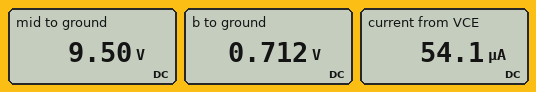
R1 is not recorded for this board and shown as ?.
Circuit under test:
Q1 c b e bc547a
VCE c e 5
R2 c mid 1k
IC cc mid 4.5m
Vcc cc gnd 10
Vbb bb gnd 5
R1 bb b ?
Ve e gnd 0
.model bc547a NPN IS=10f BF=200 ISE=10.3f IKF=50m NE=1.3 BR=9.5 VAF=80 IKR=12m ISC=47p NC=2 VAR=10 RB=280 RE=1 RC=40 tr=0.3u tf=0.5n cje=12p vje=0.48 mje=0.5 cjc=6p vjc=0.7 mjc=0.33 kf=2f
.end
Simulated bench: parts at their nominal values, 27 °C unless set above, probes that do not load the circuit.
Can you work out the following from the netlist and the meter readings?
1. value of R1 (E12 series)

120 kΩ
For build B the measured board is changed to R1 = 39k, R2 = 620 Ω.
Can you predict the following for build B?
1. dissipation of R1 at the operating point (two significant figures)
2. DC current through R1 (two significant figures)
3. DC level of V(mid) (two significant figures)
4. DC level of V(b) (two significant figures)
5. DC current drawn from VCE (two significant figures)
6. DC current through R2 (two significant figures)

460 µW
110 µA
7.8 V
770 mV
8.3 mA
4.5 mA
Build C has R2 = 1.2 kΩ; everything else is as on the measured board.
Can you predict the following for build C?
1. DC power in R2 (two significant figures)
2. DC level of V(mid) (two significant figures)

24 mW
10 V
